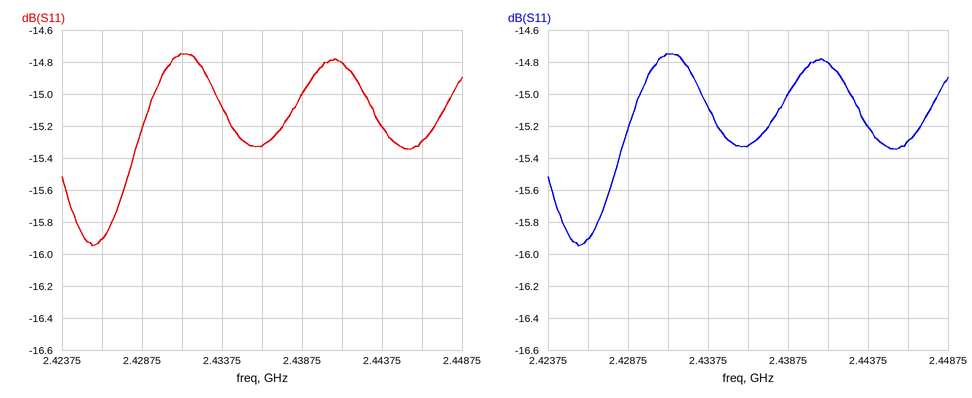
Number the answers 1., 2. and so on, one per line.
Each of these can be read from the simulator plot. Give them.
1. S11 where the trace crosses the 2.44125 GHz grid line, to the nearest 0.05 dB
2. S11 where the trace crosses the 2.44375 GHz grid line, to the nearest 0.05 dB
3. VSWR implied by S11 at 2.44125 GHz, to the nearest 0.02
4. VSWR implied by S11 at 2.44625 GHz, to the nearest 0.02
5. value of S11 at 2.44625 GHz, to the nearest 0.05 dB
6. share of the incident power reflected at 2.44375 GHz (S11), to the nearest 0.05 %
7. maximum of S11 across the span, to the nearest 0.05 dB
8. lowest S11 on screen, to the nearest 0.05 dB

1. -14.80 dB
2. -15.20 dB
3. 1.44
4. 1.42
5. -15.30 dB
6. 3.00 %
7. -14.75 dB
8. -15.95 dB
